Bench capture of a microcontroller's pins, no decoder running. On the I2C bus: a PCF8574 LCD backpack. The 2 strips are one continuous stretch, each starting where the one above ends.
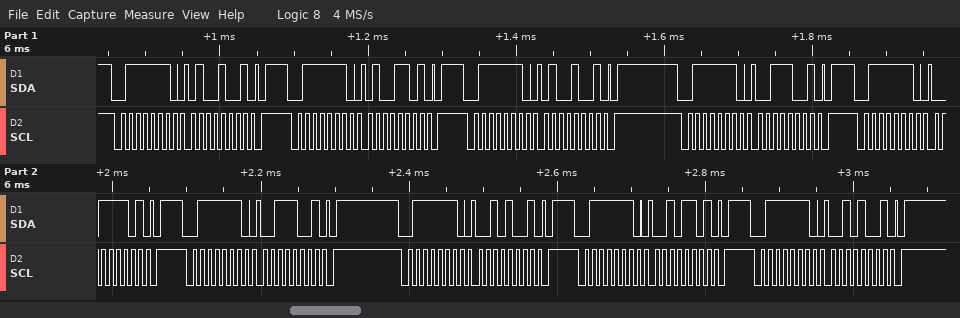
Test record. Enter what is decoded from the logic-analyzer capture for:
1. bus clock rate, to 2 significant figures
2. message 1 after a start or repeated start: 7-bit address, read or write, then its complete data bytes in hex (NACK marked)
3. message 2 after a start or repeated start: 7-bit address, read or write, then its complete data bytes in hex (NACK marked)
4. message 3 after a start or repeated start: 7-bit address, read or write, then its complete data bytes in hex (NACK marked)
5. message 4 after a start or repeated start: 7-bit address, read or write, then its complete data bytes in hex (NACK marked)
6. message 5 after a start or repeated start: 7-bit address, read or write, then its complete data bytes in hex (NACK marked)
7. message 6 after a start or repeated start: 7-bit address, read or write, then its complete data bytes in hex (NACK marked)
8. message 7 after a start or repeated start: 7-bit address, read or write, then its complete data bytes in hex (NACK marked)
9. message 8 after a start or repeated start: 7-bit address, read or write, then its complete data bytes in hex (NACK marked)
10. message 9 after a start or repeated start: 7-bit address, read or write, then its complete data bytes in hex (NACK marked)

100 kHz
0x3F write: 49
0x3F write: 4D
0x3F write: 49
0x3F write: 39
0x3F write: 3D
0x3F write: 39
0x3F write: 29
0x3F write: 2D
0x3F write: 29
